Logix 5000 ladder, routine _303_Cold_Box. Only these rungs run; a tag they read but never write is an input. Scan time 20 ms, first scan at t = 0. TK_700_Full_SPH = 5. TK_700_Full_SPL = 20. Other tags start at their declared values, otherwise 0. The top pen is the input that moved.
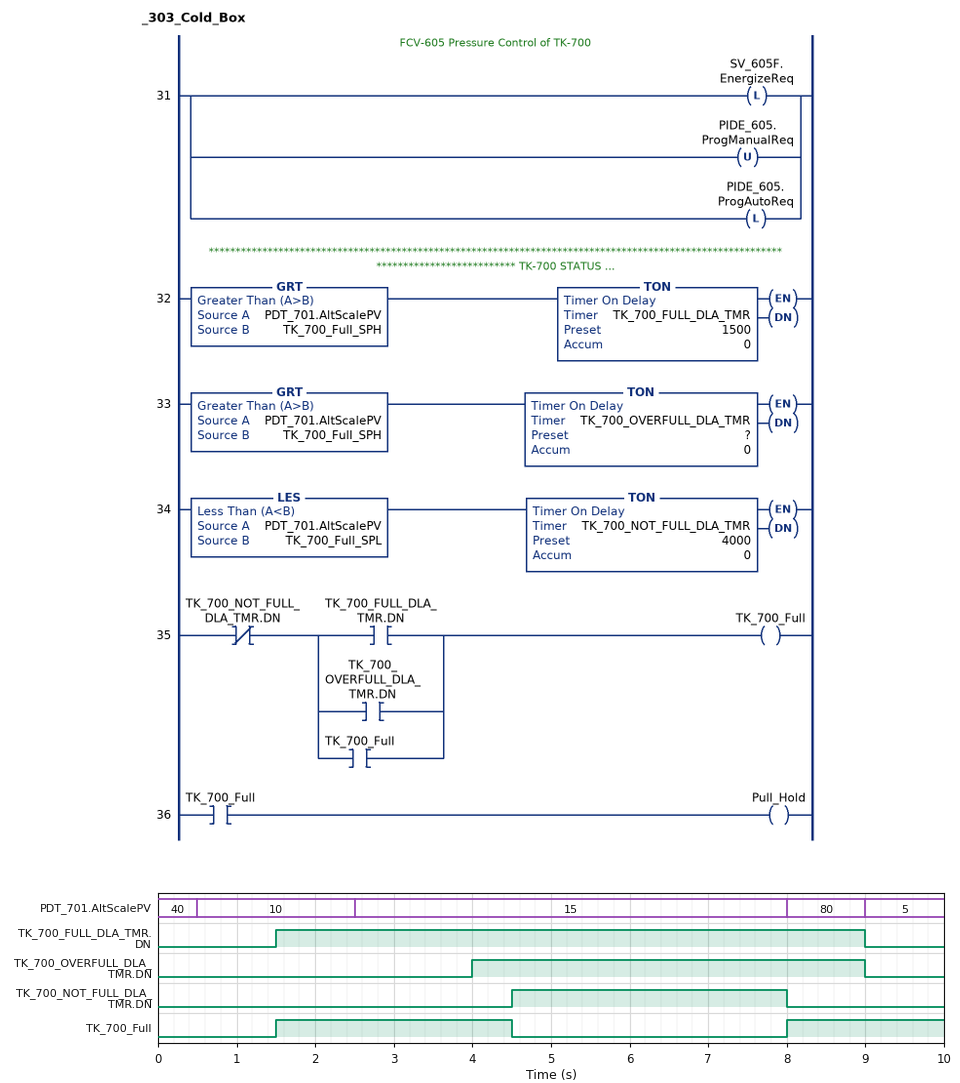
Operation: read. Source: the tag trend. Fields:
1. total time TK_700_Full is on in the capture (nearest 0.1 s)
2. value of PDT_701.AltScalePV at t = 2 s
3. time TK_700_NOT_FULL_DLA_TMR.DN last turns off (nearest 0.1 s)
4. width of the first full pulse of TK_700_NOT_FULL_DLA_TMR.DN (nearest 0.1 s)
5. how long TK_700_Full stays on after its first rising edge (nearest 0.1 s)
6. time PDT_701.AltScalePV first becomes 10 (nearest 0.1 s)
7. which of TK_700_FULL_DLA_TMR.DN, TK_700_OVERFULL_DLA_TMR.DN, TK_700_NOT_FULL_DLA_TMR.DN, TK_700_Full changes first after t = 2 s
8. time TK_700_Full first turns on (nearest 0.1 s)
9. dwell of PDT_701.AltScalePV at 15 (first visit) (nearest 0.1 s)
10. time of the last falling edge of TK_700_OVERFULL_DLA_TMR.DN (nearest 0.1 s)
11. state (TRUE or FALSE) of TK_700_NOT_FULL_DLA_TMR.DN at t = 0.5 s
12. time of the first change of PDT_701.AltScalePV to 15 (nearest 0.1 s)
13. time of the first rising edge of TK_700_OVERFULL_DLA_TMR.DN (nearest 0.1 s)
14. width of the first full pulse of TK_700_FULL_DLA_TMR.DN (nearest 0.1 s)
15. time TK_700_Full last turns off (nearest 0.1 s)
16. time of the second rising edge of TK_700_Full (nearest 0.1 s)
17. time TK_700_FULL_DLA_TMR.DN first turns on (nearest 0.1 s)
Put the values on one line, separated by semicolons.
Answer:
5.0 s; 10; 8.0 s; 3.5 s; 3.0 s; 0.5 s; TK_700_OVERFULL_DLA_TMR.DN; 1.5 s; 5.5 s; 9.0 s; FALSE; 2.5 s; 4.0 s; 7.5 s; 4.5 s; 8.0 s; 1.5 s
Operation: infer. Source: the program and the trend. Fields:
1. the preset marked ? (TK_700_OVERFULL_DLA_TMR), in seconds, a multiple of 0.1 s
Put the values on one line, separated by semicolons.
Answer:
4.0 s
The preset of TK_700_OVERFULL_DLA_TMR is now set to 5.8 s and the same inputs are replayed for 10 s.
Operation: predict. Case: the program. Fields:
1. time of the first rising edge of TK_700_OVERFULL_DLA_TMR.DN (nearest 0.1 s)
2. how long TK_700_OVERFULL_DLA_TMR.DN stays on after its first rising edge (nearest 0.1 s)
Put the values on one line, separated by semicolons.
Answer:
5.8 s; 3.2 s
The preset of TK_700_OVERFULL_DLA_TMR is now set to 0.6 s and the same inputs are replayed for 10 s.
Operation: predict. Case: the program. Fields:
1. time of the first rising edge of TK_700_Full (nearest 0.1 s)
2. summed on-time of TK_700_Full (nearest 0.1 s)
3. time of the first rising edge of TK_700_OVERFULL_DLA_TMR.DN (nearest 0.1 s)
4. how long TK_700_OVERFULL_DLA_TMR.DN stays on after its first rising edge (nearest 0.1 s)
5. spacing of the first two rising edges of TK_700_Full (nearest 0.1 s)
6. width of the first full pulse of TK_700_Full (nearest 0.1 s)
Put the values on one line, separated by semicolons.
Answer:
0.6 s; 5.9 s; 0.6 s; 8.4 s; 7.4 s; 3.9 s
